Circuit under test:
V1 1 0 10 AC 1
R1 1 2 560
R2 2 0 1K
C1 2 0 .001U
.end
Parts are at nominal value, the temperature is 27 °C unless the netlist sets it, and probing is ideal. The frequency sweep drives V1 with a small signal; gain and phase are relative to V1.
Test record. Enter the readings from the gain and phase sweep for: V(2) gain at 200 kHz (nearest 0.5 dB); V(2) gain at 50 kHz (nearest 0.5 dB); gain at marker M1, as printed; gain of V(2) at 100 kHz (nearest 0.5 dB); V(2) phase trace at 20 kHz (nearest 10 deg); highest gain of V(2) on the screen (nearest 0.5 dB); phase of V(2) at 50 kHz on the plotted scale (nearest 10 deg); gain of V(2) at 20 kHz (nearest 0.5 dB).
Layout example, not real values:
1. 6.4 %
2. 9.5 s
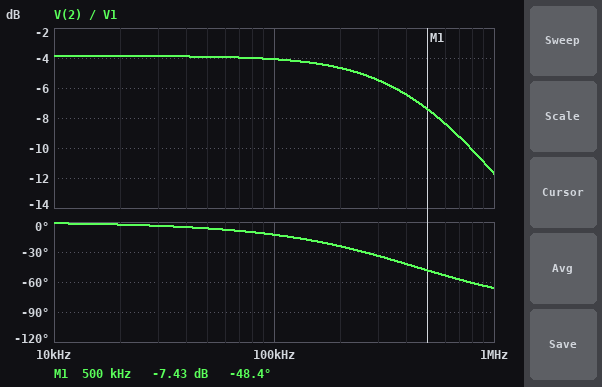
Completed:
1. -4.5 dB
2. -4.0 dB
3. -7.43 dB
4. -4.0 dB
5. 0 deg
6. -4.0 dB
7. -10 deg
8. -4.0 dB
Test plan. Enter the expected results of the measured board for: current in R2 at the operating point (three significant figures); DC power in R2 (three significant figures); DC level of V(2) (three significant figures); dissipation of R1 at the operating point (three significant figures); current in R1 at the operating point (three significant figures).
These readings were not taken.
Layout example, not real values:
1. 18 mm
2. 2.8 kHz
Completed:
1. 6.41 mA
2. 41.1 mW
3. 6.41 V
4. 23.0 mW
5. 6.41 mA
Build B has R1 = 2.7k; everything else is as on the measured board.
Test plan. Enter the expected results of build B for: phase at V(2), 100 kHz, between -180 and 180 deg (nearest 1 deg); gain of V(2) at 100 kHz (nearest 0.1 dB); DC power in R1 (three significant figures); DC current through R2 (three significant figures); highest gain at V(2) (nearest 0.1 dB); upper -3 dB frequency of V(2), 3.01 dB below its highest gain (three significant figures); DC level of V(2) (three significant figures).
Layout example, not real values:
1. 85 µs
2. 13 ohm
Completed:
1. -25 deg
2. -12.2 dB
3. 19.7 mW
4. 2.70 mA
5. -11.4 dB
6. 218 kHz
7. 2.70 V
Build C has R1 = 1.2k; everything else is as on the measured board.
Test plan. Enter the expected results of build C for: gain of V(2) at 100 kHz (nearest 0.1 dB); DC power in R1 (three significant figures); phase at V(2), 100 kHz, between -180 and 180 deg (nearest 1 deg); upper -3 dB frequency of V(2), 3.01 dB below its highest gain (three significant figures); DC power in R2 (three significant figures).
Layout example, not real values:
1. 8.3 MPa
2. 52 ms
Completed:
1. -7.3 dB
2. 24.8 mW
3. -19 deg
4. 292 kHz
5. 20.7 mW
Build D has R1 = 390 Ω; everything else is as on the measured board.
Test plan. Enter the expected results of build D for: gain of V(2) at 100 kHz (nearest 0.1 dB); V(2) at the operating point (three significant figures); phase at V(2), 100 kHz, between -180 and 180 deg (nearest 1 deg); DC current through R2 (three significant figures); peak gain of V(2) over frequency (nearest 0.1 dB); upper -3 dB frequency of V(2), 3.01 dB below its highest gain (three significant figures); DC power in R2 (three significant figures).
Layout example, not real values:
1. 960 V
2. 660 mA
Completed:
1. -3.0 dB
2. 7.19 V
3. -10 deg
4. 7.19 mA
5. -2.9 dB
6. 567 kHz
7. 51.8 mW
